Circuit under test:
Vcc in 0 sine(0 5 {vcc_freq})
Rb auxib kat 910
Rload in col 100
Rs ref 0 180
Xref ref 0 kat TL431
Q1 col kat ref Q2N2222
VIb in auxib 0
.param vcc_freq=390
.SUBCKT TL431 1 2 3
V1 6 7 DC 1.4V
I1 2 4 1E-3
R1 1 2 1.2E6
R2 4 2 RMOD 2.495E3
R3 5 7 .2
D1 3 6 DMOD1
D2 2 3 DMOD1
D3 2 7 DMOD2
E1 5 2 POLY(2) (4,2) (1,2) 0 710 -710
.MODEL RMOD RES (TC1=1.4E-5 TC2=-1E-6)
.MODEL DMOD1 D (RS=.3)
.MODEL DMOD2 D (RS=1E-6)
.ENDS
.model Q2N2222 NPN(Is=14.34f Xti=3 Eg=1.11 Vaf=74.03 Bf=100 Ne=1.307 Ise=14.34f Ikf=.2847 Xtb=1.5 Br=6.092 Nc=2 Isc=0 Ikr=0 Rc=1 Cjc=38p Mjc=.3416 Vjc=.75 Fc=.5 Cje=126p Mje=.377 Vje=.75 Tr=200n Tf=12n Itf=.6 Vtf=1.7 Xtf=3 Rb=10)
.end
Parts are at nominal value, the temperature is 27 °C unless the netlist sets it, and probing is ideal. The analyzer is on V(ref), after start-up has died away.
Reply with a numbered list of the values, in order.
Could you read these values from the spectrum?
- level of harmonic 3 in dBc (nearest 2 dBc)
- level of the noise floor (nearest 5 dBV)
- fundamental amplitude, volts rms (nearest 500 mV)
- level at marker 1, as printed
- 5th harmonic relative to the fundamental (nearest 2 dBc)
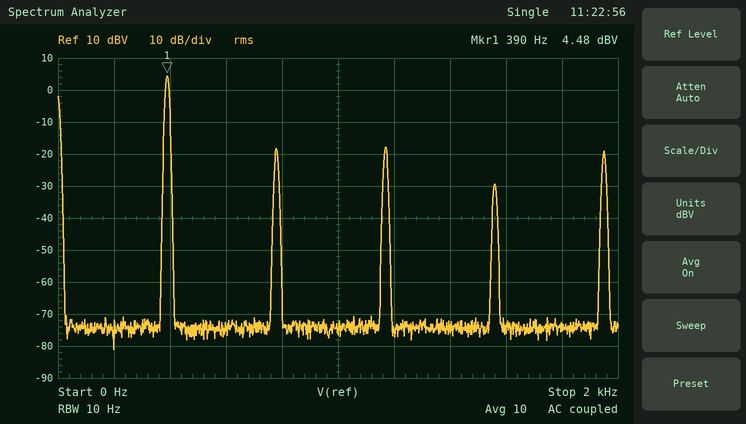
1. -22 dBc
2. -75 dBV
3. 1.5 V
4. 4.48 dBV
5. -24 dBc
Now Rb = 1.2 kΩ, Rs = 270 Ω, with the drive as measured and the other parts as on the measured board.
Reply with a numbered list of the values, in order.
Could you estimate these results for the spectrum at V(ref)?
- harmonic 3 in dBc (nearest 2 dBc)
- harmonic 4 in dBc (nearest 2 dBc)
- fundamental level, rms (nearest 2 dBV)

1. -20 dBc
2. -30 dBc
3. 4 dBV
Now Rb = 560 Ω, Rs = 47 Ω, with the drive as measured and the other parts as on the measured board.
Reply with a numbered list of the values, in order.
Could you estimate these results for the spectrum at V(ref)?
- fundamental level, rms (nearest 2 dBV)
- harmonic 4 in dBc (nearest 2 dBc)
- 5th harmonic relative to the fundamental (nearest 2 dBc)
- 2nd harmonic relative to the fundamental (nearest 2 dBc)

1. 0 dBV
2. -30 dBc
3. -28 dBc
4. -36 dBc
